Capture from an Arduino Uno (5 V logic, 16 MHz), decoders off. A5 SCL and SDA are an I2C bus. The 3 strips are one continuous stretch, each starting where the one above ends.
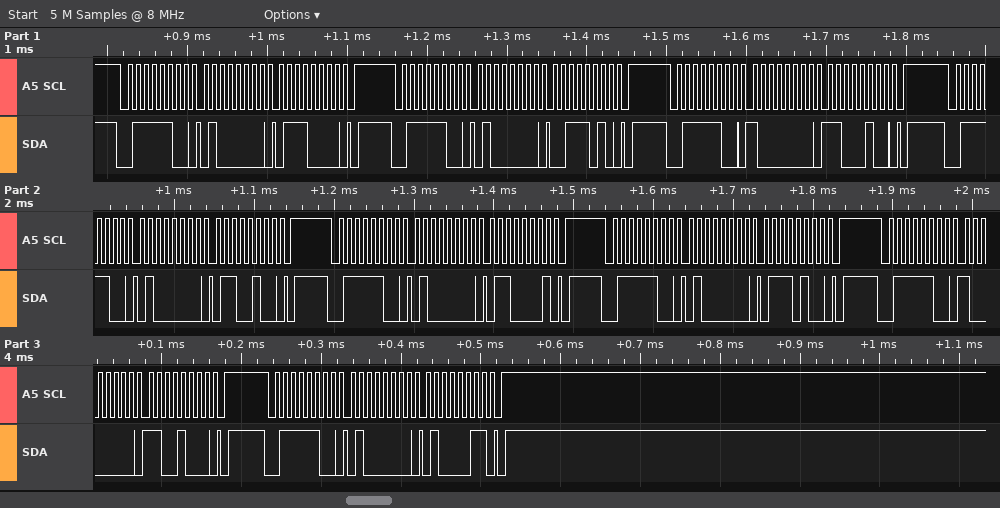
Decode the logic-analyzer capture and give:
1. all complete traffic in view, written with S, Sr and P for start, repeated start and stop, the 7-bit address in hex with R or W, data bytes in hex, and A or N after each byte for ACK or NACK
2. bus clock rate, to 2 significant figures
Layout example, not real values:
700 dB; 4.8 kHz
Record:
S 3EW A 40 A 70 A P S 3EW A 40 A 3A A P S 3EW A 80 A C4 A P S 3EW A 40 A 64 A P S 3EW A 40 A 61 A P S 3EW A 40 A 74 A P S 3EW A 80 A C8 A P S 3EW A 40 A 43 A P; 100 kHz
